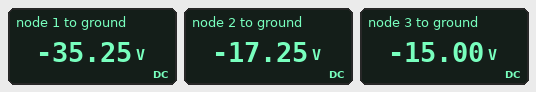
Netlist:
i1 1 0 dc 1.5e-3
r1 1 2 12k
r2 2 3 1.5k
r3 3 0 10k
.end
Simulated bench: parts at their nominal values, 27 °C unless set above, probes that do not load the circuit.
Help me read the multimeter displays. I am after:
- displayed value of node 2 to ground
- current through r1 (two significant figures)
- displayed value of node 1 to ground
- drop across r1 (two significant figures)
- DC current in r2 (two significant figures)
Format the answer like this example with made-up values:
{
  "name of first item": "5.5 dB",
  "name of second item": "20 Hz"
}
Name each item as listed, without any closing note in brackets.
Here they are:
{
  "displayed value of node 2 to ground": "-17.25 V",
  "current through r1": "1.5 mA",
  "displayed value of node 1 to ground": "-35.25 V",
  "drop across r1": "18 V",
  "DC current in r2": "1.5 mA"
}
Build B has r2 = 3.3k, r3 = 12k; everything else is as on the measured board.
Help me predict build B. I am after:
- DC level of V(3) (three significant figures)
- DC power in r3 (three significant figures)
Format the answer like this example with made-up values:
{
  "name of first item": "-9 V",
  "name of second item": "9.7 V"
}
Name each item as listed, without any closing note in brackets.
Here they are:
{
  "DC level of V(3)": "-18.0 V",
  "DC power in r3": "27.0 mW"
}
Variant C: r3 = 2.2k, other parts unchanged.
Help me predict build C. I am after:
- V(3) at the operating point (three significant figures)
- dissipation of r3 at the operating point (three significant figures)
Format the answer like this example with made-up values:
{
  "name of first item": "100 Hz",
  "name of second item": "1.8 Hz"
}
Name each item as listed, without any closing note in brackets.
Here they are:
{
  "V(3) at the operating point": "-3.30 V",
  "dissipation of r3 at the operating point": "4.95 mW"
}
